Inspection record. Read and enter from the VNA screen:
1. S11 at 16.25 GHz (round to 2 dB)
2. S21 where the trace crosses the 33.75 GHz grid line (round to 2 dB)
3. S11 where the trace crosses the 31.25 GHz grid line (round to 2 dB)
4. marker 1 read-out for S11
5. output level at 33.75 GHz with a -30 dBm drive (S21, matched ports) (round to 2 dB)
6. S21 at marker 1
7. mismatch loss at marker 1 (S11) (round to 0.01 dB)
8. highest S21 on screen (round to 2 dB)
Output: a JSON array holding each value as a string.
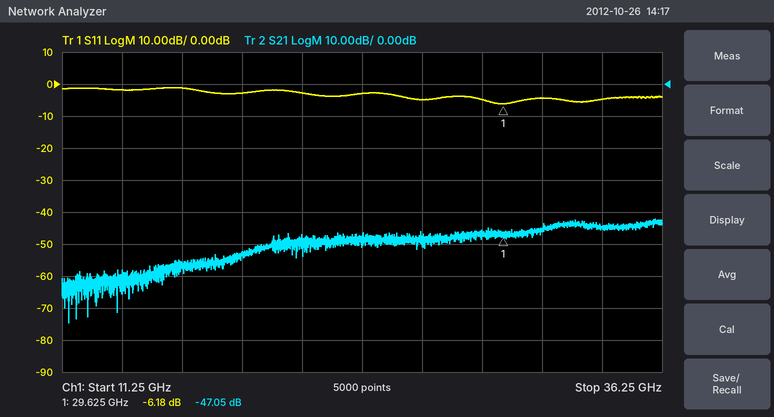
["-2 dB", "-44 dB", "-4 dB", "-6.18 dB", "-74 dBm", "-47.05 dB", "1.20 dB", "-42 dB"]
